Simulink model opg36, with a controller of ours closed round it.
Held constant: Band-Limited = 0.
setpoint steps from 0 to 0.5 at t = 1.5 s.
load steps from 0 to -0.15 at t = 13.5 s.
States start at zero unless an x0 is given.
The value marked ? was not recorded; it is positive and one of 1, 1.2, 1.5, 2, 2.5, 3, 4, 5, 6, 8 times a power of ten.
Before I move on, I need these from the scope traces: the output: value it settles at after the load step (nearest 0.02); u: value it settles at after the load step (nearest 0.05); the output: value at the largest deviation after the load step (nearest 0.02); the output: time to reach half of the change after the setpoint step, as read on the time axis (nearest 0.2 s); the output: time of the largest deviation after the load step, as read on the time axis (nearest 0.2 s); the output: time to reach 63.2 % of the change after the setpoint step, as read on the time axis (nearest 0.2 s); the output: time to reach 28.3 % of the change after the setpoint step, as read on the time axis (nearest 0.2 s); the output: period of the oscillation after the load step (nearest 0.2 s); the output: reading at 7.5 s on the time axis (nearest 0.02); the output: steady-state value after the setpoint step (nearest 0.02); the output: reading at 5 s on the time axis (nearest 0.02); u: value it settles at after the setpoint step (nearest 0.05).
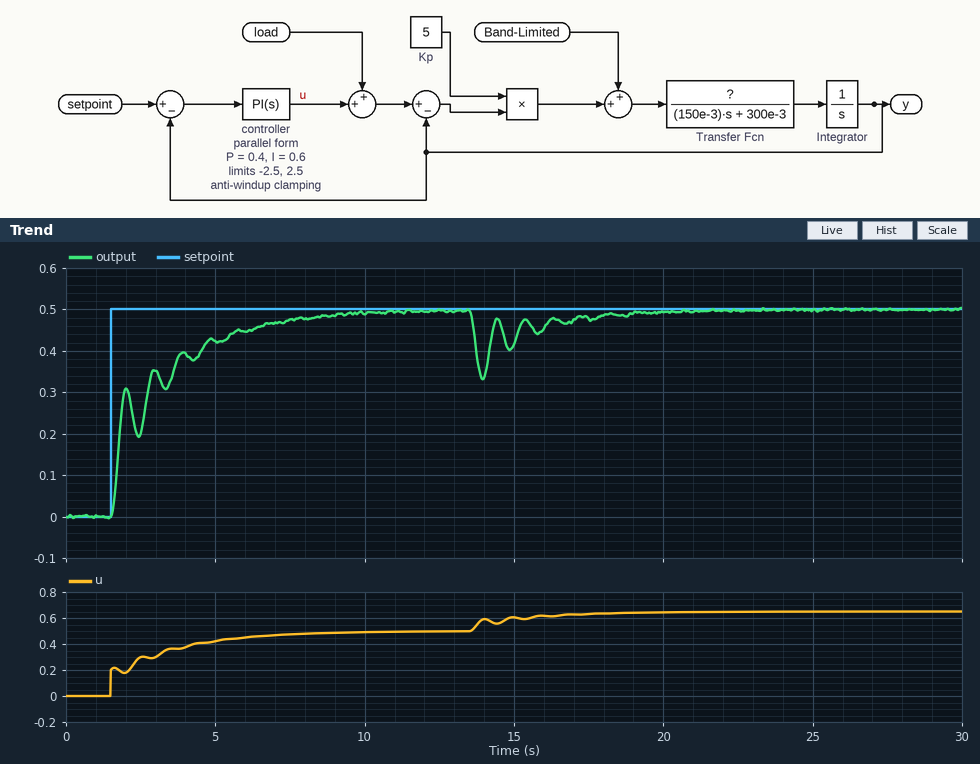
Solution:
0.50
0.65
0.34
1.8 s
14.0 s
2.8 s
1.8 s
1.0 s
0.48
0.50
0.42
0.50
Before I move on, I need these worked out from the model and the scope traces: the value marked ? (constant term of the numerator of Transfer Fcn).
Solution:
1
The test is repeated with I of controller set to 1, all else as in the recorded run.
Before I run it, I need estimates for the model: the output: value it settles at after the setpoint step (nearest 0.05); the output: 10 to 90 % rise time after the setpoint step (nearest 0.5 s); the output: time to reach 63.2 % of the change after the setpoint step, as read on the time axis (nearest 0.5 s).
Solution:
0.50
2.0 s
2.0 s
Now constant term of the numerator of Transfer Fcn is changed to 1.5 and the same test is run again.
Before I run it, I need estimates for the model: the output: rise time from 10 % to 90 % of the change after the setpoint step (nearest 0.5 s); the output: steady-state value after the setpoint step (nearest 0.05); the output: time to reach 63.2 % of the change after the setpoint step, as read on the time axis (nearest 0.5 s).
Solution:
4.5 s
0.50
2.5 s
